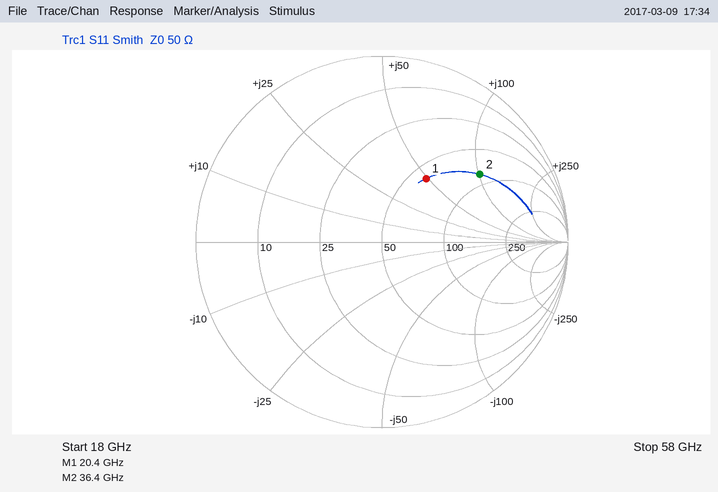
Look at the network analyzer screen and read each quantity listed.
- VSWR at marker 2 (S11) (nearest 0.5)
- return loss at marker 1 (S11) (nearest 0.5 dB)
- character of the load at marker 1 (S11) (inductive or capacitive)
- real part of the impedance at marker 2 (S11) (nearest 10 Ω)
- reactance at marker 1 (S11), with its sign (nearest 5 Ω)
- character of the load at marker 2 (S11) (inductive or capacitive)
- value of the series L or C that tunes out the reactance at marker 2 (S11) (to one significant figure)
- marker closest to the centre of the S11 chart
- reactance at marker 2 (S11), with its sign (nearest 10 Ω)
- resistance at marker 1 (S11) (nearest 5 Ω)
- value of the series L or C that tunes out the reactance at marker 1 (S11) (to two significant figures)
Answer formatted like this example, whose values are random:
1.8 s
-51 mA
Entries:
4.5
7.5 dB
inductive
80 Ω
+50 Ω
inductive
40 fF
marker 1
+100 Ω
60 Ω
160 fF
